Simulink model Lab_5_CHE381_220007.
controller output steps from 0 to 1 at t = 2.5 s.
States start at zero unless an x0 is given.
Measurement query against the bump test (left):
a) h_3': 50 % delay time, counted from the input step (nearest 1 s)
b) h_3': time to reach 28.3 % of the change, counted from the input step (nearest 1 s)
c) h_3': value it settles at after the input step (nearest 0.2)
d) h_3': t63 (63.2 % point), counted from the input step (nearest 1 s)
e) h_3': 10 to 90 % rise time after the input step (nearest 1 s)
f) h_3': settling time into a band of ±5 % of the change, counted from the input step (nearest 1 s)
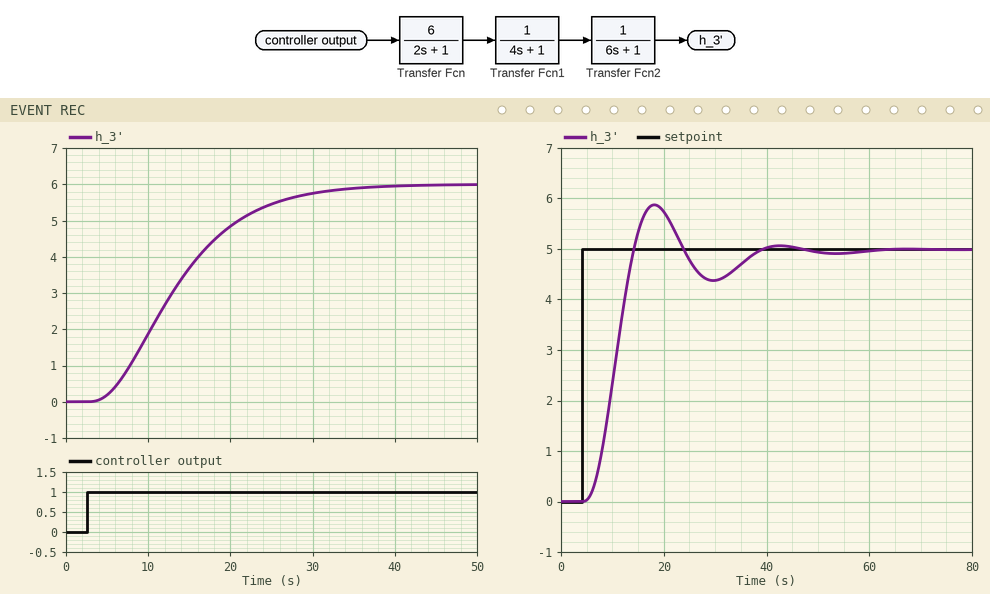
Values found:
10 s
7 s
6.0
13 s
18 s
26 s
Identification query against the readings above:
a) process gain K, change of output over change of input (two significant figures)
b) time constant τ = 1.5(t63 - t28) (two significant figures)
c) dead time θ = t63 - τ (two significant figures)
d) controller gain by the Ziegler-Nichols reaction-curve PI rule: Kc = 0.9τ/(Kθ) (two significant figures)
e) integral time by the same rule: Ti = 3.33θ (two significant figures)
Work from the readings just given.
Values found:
6.0
9.0 s
4.0 s
0.34
13 s
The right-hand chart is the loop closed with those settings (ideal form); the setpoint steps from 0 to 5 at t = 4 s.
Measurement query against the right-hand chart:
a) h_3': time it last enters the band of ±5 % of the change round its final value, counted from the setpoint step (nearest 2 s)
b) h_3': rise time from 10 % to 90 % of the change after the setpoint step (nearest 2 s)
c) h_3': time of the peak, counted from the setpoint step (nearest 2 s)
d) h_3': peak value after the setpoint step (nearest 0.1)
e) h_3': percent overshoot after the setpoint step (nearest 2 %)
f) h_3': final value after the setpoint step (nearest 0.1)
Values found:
32 s
6 s
14 s
5.9
18 %
5.0
